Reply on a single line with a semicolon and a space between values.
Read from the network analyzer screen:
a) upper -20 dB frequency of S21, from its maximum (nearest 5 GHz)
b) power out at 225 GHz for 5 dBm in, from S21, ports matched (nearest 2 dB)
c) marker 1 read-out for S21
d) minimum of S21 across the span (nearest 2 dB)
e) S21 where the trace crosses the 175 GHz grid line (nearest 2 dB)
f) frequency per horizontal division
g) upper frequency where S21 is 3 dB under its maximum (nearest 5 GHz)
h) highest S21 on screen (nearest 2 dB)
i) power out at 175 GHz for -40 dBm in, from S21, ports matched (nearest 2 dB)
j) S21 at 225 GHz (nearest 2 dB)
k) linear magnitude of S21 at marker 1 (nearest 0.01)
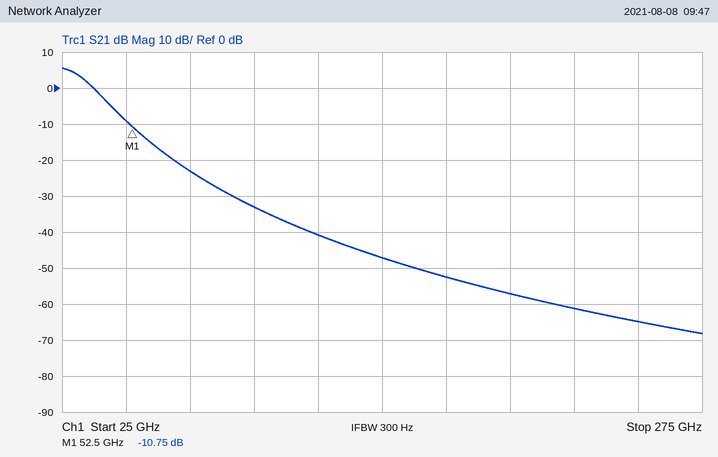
60 GHz; -56 dBm; -10.75 dB; -68 dB; -52 dB; 25 GHz; 35 GHz; 6 dB; -92 dBm; -62 dB; 0.29
